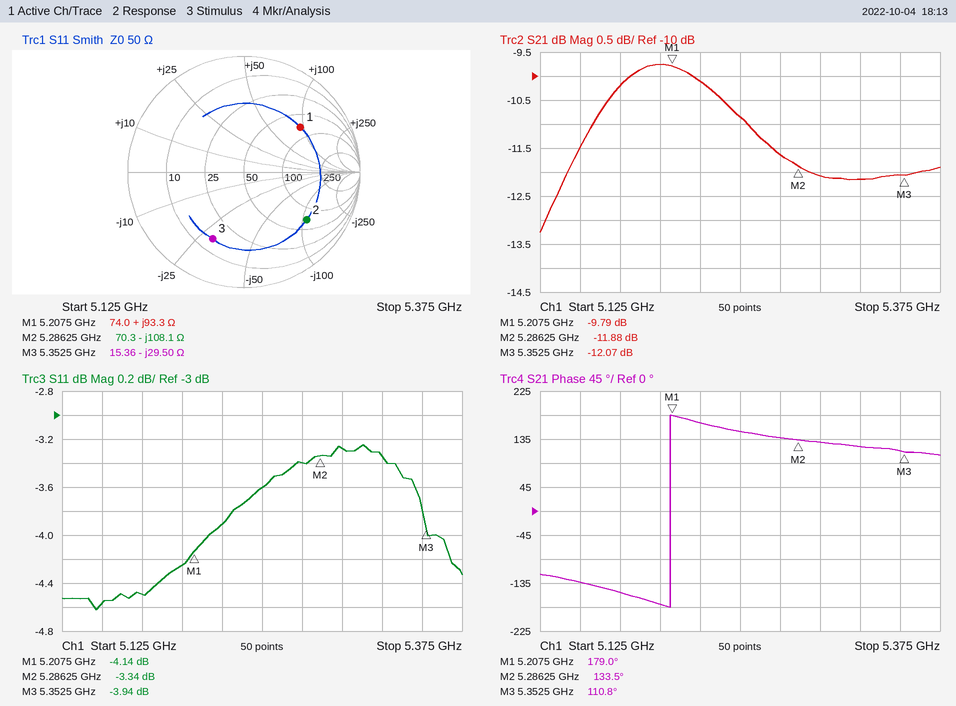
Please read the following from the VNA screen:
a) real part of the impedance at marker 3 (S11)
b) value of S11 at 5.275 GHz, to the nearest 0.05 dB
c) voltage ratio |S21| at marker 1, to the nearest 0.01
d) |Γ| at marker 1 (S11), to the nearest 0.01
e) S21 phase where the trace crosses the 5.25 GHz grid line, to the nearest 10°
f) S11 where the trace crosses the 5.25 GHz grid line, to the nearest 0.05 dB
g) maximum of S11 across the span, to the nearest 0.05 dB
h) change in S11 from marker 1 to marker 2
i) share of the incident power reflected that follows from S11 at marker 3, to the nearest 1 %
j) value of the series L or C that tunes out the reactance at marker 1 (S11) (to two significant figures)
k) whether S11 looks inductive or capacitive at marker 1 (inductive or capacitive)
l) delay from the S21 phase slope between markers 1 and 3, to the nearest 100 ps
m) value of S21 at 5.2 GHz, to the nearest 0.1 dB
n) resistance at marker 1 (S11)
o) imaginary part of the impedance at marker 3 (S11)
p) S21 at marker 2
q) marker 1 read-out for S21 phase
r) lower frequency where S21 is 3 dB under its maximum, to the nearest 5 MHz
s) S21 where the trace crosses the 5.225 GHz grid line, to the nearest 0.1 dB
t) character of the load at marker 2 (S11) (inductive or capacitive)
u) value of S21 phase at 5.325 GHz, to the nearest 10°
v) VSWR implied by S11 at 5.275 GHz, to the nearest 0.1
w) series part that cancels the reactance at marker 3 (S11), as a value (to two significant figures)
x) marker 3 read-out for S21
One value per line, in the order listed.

15.36 Ω
-3.40 dB
0.32
0.62
150°
-3.60 dB
-3.25 dB
0.80 dB
40 %
330 fF
inductive
1.3 ns
-9.8 dB
74.0 Ω
-29.50 Ω
-11.88 dB
179.0°
5.130 GHz
-10.1 dB
capacitive
120°
5.2
880 pH
-12.07 dB
